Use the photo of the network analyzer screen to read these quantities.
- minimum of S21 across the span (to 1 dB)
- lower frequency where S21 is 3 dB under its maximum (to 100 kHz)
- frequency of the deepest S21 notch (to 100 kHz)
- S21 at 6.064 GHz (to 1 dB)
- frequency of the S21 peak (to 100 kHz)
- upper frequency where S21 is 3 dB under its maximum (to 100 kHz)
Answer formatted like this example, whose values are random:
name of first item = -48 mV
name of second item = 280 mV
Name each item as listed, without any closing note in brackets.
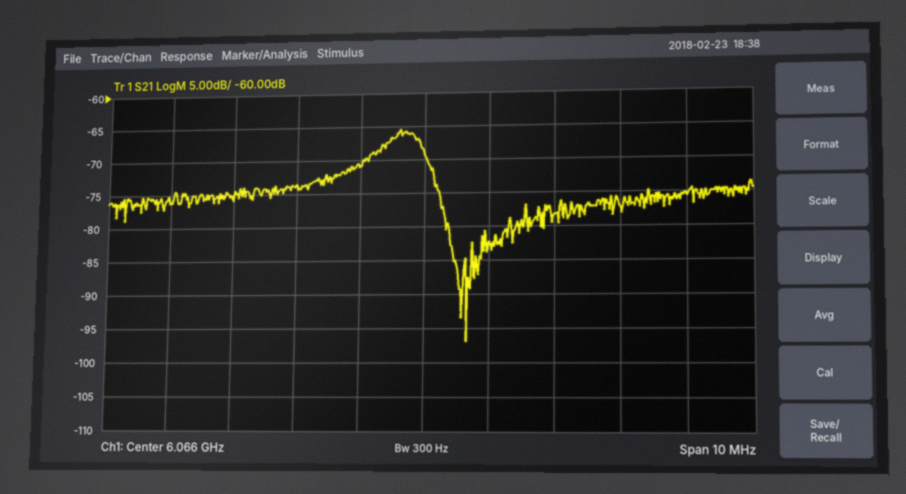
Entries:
minimum of S21 across the span = -97 dB
lower frequency where S21 is 3 dB under its maximum = 6.0653 GHz
frequency of the deepest S21 notch = 6.0667 GHz
S21 at 6.064 GHz = -74 dB
frequency of the S21 peak = 6.0656 GHz
upper frequency where S21 is 3 dB under its maximum = 6.0660 GHz
